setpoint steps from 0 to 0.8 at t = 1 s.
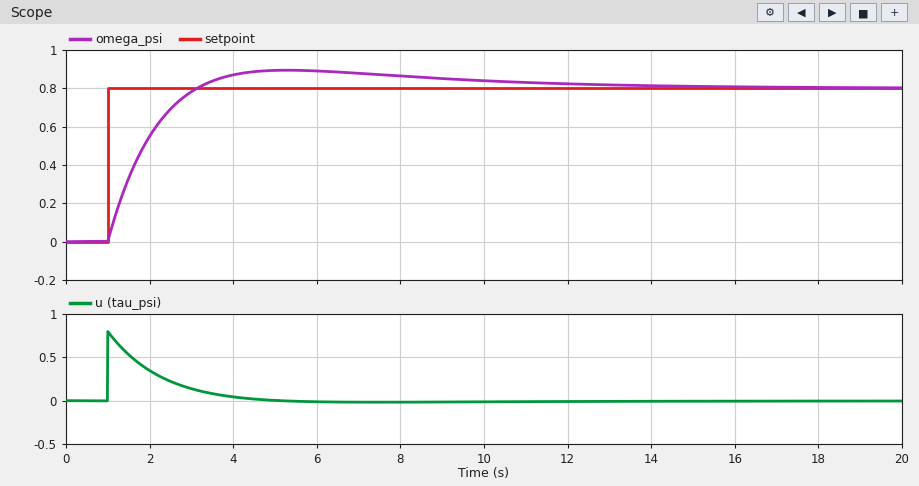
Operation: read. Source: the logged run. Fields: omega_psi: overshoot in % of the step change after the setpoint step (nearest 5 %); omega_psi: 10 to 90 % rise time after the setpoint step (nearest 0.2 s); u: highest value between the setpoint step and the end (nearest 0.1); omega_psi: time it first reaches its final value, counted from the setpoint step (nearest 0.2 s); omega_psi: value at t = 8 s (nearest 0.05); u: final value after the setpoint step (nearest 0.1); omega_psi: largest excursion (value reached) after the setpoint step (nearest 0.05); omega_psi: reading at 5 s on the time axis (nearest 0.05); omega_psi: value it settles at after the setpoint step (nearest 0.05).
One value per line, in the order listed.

10 %
1.6 s
0.8
2.2 s
0.85
0.0
0.90
0.90
0.80
